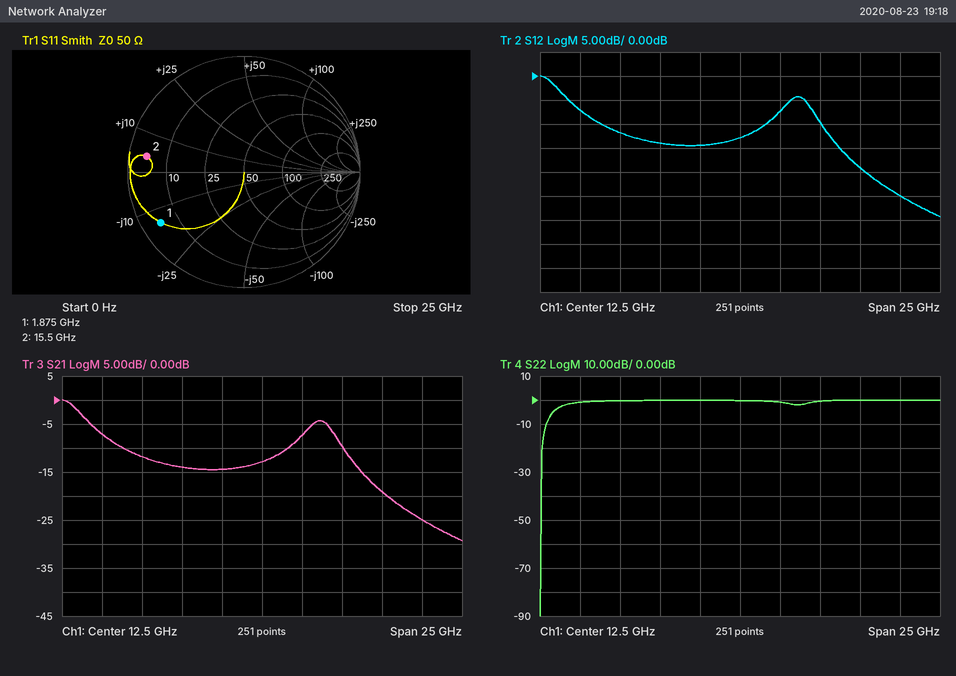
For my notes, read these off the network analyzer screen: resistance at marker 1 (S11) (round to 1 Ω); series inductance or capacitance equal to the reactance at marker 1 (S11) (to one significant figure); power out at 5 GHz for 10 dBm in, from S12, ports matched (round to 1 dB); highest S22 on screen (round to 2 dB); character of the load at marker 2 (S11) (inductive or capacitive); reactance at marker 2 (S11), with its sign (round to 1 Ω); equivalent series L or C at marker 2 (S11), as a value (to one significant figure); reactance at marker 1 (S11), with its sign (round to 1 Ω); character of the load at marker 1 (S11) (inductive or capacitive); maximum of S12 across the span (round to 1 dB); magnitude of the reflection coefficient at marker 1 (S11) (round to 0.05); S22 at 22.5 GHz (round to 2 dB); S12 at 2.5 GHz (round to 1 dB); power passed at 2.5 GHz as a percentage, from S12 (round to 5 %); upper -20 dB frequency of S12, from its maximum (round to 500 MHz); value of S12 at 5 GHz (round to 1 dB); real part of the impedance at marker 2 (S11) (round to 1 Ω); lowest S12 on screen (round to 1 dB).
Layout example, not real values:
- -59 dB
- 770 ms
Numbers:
- 5 Ω
- 6 pF
- -2 dBm
- 0 dB
- inductive
- +4 Ω
- 40 pH
- -14 Ω
- capacitive
- 0 dB
- 0.85
- 0 dB
- -7 dB
- 20 %
- 20.5 GHz
- -12 dB
- 4 Ω
- -29 dB
